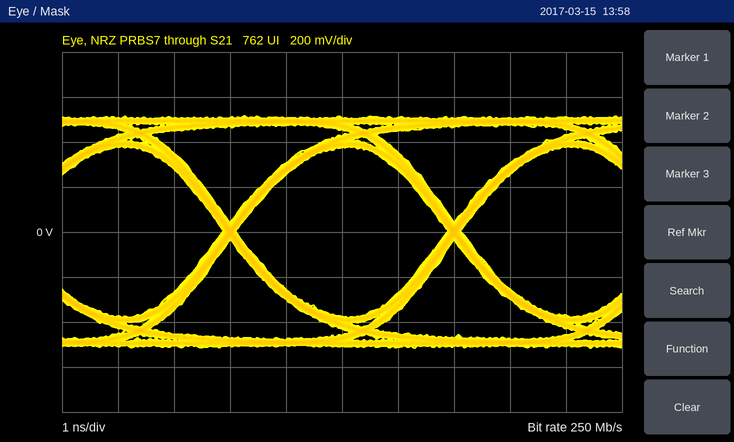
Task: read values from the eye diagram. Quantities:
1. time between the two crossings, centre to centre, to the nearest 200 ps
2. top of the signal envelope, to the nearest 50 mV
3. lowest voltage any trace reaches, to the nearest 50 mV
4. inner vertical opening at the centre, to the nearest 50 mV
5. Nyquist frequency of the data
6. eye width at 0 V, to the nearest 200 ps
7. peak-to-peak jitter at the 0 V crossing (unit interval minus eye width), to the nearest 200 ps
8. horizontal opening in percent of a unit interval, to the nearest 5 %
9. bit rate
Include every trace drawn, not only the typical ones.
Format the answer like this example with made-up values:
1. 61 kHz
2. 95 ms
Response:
1. 4.0 ns
2. 500 mV
3. -500 mV
4. 750 mV
5. 125 MHz
6. 3.8 ns
7. 200 ps
8. 95 %
9. 250 Mb/s
